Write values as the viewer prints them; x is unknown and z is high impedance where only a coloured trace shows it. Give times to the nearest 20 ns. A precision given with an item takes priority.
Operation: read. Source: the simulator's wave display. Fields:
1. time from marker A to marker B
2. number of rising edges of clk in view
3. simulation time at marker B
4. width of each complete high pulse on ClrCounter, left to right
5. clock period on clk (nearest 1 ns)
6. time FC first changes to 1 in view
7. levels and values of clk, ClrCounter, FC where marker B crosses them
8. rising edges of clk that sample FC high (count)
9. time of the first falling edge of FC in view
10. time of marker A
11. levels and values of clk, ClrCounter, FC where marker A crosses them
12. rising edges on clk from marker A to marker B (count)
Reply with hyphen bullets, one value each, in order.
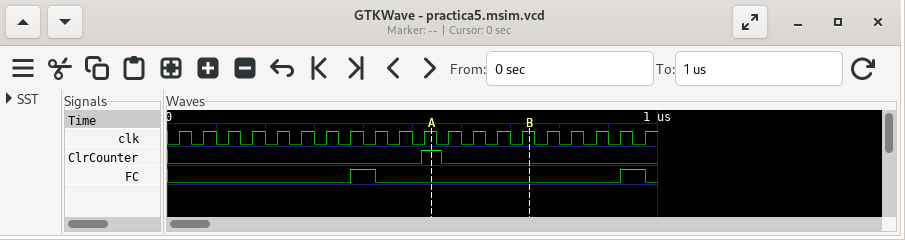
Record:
- 200 ns
- 20
- 740 ns
- 40 ns
- 50 ns
- 380 ns
- clk=1, ClrCounter=0, FC=0
- 2
- 420 ns
- 540 ns
- clk=1, ClrCounter=1, FC=0
- 4
